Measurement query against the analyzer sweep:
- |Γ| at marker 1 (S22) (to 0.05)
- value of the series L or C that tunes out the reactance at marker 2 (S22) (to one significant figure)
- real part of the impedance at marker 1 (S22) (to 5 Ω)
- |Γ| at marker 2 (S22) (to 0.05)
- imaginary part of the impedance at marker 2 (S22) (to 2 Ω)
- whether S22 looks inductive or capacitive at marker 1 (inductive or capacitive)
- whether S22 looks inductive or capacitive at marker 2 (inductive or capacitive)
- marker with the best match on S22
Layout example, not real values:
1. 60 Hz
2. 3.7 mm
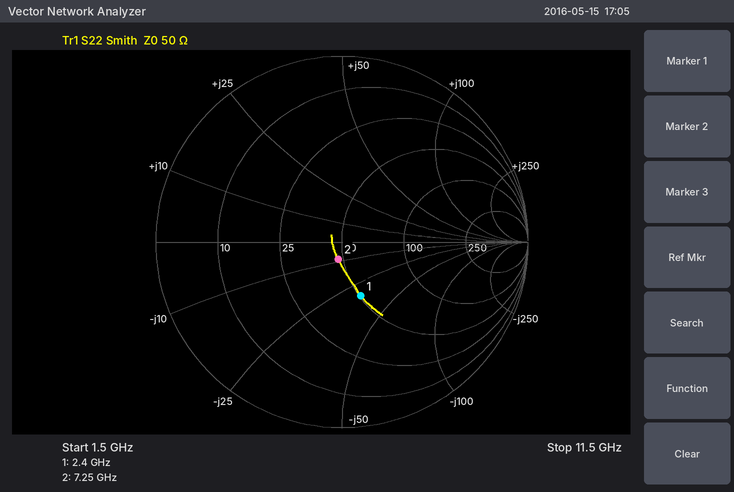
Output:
1. 0.30
2. 200 pH
3. 50 Ω
4. 0.10
5. -8 Ω
6. capacitive
7. capacitive
8. marker 2
